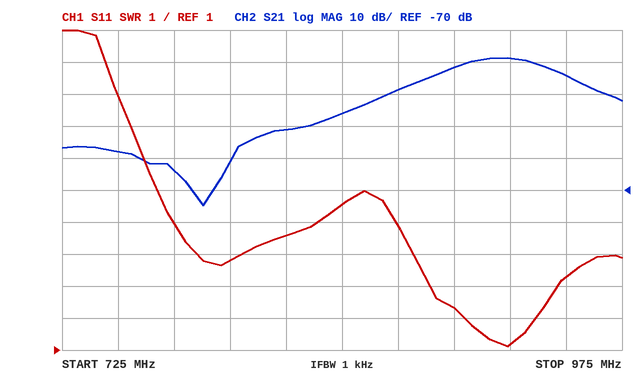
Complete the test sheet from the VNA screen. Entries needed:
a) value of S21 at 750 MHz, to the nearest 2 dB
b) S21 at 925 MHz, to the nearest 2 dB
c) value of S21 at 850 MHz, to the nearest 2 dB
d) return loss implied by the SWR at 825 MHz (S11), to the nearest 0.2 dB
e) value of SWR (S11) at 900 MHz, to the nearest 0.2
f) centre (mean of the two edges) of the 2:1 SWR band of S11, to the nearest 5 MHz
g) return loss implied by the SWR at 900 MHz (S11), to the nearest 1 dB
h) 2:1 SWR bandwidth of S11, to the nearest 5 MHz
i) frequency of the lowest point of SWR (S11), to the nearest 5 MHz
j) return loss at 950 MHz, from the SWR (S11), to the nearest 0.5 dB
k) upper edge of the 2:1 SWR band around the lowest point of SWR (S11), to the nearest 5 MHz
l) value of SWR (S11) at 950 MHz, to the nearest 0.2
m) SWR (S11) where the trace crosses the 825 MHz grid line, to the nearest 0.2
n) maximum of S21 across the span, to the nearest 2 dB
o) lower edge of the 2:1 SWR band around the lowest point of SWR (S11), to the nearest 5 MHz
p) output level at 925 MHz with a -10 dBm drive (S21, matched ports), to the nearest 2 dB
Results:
-58 dB
-28 dB
-46 dB
3.8 dB
2.4
920 MHz
8 dB
30 MHz
925 MHz
5.5 dB
935 MHz
3.2
4.6
-28 dB
905 MHz
-38 dBm
